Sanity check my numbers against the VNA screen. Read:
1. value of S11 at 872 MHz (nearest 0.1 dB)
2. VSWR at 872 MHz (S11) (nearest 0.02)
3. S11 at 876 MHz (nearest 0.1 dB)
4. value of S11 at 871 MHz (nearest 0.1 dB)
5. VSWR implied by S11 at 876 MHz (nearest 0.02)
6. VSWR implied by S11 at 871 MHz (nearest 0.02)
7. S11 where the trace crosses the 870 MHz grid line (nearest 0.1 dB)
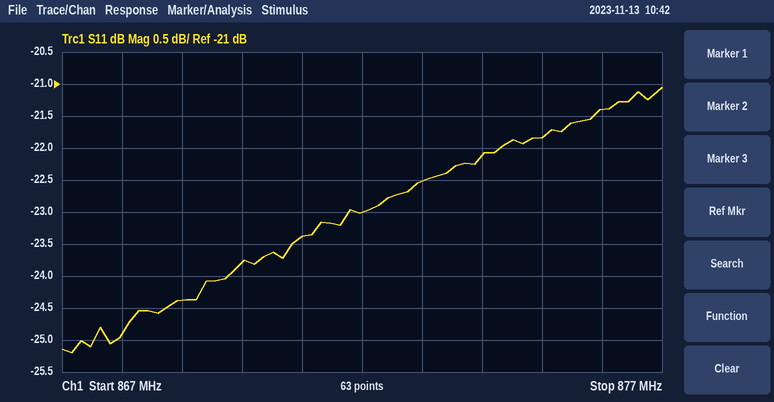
-23.0 dB
1.16
-21.4 dB
-23.4 dB
1.18
1.14
-23.8 dB
